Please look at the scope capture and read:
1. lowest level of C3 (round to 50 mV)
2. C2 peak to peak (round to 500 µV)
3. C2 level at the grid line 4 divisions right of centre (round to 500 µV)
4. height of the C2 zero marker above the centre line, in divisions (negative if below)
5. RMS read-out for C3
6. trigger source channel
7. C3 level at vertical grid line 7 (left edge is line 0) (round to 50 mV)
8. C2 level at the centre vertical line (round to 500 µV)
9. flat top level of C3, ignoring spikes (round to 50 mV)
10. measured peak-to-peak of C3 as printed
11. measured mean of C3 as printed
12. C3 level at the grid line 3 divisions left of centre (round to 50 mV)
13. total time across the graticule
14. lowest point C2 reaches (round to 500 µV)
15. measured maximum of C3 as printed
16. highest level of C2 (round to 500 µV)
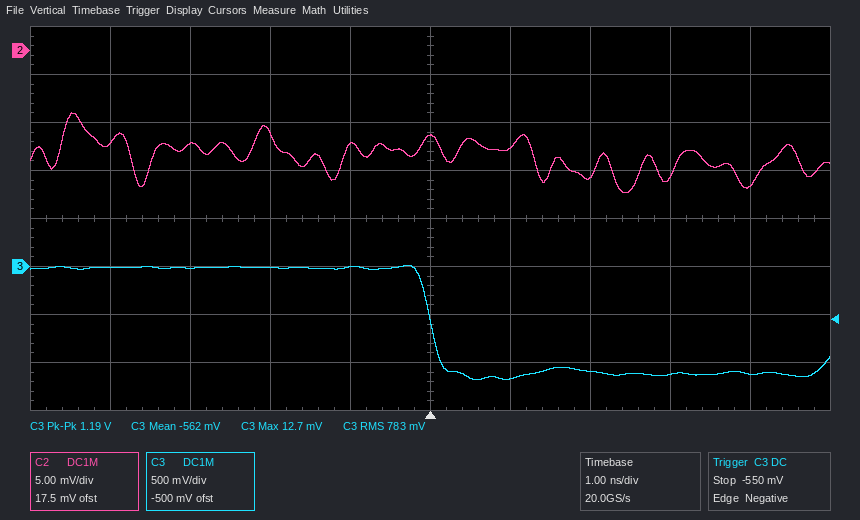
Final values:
-1.20 V
8.5 mV
-14.0 mV
+3.5 div
783 mV
C3
-1.10 V
-9.0 mV
0 mV
1.19 V
-562 mV
0 mV
10 ns
-15.0 mV
12.7 mV
-6.5 mV
